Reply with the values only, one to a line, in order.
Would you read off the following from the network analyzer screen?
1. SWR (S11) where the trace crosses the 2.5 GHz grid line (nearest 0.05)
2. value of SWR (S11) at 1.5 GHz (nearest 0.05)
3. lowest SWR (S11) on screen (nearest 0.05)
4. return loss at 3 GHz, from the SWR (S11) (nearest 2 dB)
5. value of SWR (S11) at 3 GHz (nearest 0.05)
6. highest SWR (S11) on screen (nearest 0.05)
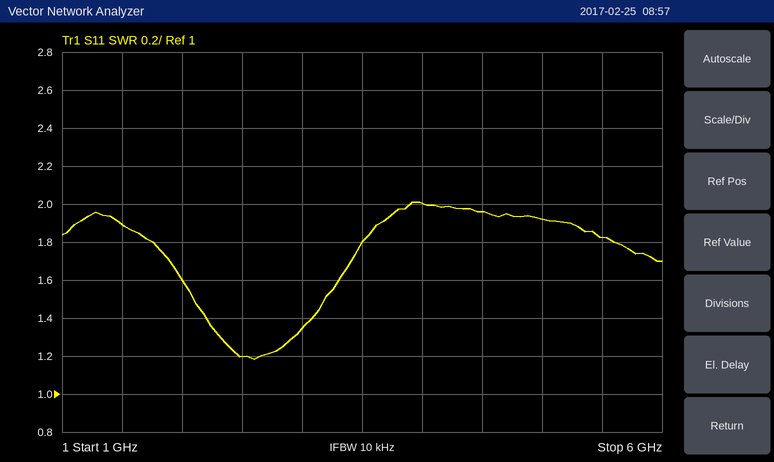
1.20
1.90
1.20
16 dB
1.35
2.00
